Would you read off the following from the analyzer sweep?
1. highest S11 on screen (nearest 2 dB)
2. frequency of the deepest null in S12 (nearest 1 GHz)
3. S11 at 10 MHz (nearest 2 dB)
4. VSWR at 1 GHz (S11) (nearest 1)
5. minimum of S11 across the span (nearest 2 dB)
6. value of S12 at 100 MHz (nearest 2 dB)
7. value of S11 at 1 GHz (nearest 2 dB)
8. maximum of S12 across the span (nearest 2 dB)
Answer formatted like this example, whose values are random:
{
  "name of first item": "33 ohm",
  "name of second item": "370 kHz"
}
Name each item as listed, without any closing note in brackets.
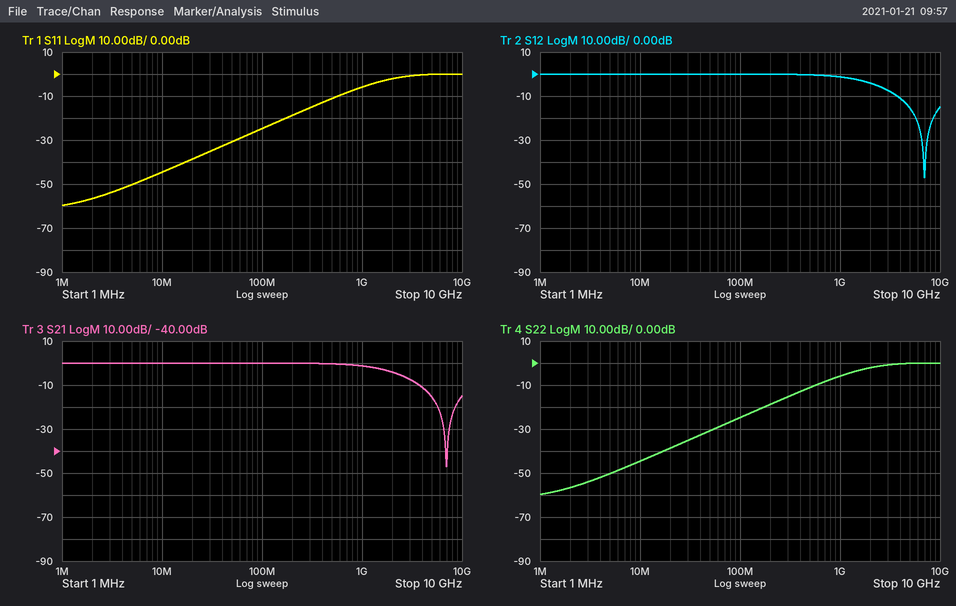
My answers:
{
  "highest S11 on screen": "0 dB",
  "frequency of the deepest null in S12": "7 GHz",
  "S11 at 10 MHz": "-44 dB",
  "VSWR at 1 GHz (S11)": "3",
  "minimum of S11 across the span": "-60 dB",
  "value of S12 at 100 MHz": "0 dB",
  "value of S11 at 1 GHz": "-6 dB",
  "maximum of S12 across the span": "0 dB"
}
